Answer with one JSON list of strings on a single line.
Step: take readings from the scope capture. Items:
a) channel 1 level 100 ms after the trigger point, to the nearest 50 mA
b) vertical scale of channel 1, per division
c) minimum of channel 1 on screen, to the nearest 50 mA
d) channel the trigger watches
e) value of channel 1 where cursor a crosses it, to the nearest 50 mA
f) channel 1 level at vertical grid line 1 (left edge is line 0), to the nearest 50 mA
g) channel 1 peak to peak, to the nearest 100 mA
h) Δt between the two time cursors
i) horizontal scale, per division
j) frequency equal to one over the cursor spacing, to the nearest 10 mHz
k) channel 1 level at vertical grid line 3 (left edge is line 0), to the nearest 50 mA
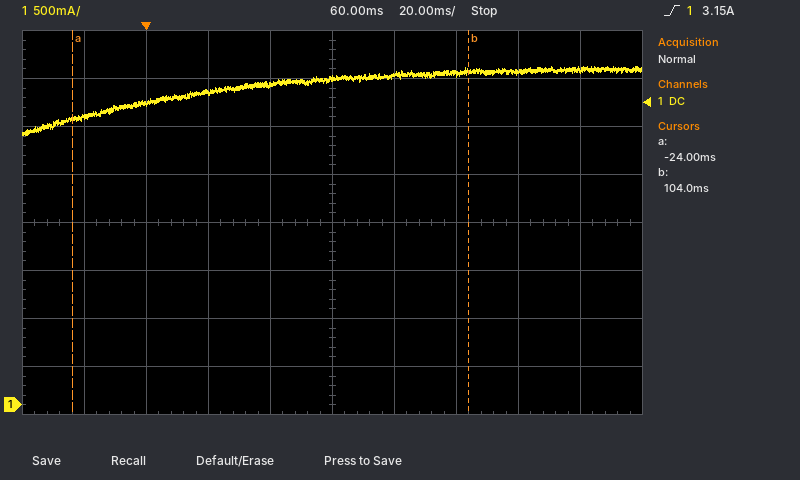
["3.45 A", "500 mA", "2.80 A", "channel 1", "3.00 A", "3.00 A", "700 mA", "128 ms", "20 ms", "7.81 Hz", "3.25 A"]
